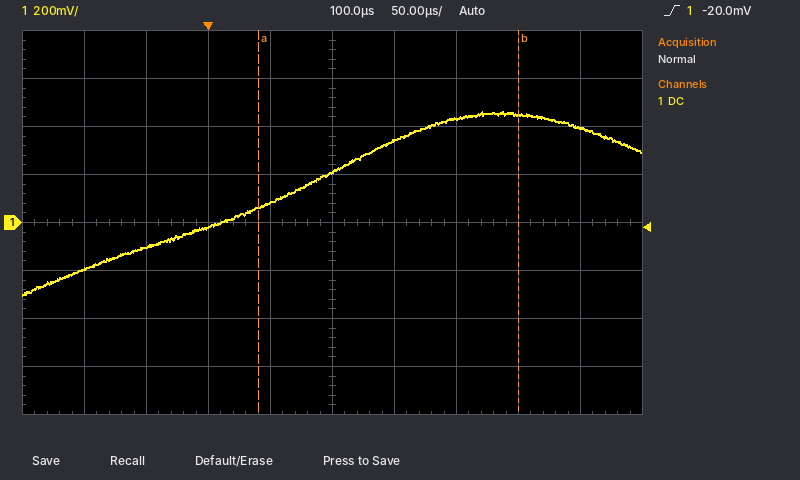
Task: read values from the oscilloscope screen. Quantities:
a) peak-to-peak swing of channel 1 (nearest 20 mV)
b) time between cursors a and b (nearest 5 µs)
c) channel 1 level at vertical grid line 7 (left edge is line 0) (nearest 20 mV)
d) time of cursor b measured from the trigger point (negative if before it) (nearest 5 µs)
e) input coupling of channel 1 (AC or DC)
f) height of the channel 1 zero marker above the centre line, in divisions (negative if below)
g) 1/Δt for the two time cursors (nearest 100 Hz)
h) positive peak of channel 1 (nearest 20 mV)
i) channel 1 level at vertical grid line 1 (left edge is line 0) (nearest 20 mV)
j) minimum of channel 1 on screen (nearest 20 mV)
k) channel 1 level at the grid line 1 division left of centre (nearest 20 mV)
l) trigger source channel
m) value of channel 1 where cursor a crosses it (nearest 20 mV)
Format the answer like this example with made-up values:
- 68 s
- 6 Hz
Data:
- 760 mV
- 210 µs
- 440 mV
- +250 µs
- DC
- 0.0 div
- 4.8 kHz
- 460 mV
- -200 mV
- -300 mV
- 80 mV
- channel 1
- 60 mV
